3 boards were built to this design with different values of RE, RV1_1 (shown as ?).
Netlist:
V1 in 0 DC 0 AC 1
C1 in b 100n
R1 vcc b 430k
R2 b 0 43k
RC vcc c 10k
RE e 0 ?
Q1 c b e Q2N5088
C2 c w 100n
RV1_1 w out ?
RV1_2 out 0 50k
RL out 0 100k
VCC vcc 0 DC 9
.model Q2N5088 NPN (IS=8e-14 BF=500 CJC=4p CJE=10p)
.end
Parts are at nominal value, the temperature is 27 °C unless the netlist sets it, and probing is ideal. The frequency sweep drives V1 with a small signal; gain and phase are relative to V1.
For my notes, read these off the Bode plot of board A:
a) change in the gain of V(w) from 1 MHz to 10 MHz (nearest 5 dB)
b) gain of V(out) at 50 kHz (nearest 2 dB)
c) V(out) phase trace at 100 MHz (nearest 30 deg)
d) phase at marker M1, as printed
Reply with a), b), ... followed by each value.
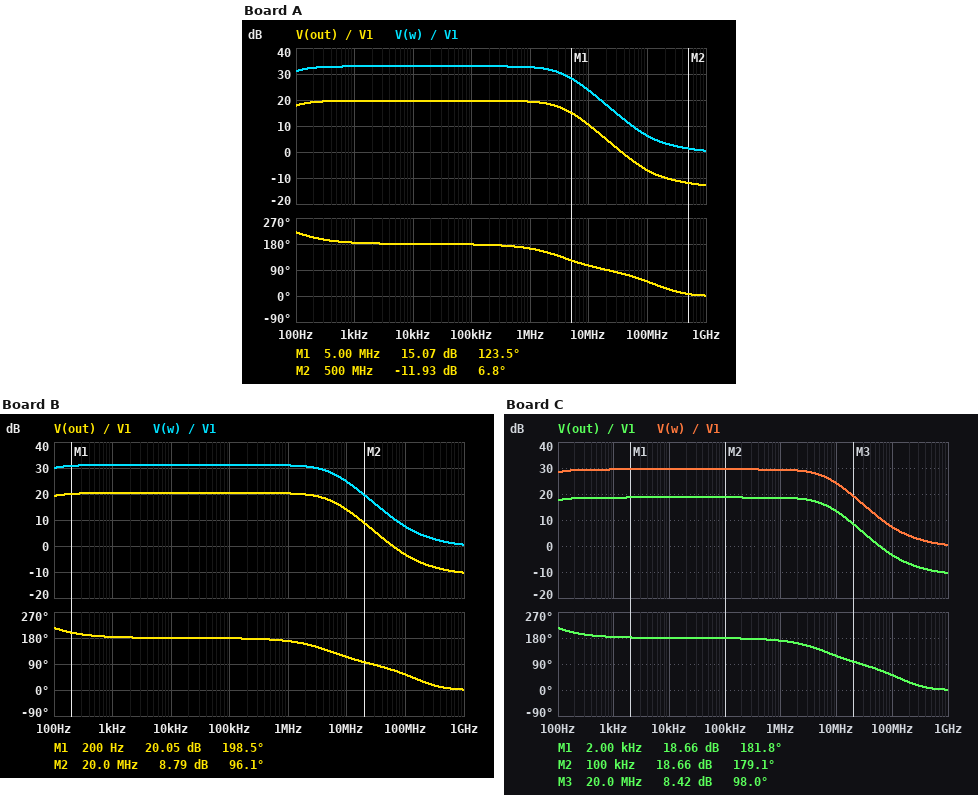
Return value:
a) -10 dB
b) 20 dB
c) 60 deg
d) 123.5 deg
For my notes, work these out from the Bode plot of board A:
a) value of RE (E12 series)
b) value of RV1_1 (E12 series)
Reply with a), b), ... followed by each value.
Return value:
a) 180 Ω
b) 120 kΩ
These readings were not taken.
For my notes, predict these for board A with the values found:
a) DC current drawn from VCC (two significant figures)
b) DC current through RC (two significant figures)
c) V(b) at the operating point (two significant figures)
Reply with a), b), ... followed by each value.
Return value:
a) 870 µA
b) 850 µA
c) 750 mV
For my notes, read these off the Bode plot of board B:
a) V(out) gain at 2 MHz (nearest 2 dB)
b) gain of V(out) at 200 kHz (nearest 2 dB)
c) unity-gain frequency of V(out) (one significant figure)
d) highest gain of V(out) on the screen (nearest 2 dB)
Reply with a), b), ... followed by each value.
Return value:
a) 20 dB
b) 20 dB
c) 60 MHz
d) 20 dB
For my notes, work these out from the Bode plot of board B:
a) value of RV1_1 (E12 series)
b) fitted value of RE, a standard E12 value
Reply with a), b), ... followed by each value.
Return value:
a) 82 kΩ
b) 220 Ω
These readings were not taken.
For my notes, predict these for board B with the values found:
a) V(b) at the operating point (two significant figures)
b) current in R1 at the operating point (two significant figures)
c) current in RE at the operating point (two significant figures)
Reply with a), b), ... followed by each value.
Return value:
a) 760 mV
b) 19 µA
c) 750 µA
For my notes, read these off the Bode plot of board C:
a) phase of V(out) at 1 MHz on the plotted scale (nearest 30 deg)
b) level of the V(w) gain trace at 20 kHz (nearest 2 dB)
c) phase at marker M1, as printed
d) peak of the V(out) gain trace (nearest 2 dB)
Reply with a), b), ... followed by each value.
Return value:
a) 180 deg
b) 30 dB
c) 181.8 deg
d) 18 dB
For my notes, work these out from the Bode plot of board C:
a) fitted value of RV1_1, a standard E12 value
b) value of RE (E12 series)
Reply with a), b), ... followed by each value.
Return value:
a) 82 kΩ
b) 270 Ω
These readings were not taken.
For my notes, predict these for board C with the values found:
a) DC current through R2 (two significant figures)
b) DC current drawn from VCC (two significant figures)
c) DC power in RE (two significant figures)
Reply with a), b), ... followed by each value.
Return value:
a) 18 µA
b) 670 µA
c) 120 µW
